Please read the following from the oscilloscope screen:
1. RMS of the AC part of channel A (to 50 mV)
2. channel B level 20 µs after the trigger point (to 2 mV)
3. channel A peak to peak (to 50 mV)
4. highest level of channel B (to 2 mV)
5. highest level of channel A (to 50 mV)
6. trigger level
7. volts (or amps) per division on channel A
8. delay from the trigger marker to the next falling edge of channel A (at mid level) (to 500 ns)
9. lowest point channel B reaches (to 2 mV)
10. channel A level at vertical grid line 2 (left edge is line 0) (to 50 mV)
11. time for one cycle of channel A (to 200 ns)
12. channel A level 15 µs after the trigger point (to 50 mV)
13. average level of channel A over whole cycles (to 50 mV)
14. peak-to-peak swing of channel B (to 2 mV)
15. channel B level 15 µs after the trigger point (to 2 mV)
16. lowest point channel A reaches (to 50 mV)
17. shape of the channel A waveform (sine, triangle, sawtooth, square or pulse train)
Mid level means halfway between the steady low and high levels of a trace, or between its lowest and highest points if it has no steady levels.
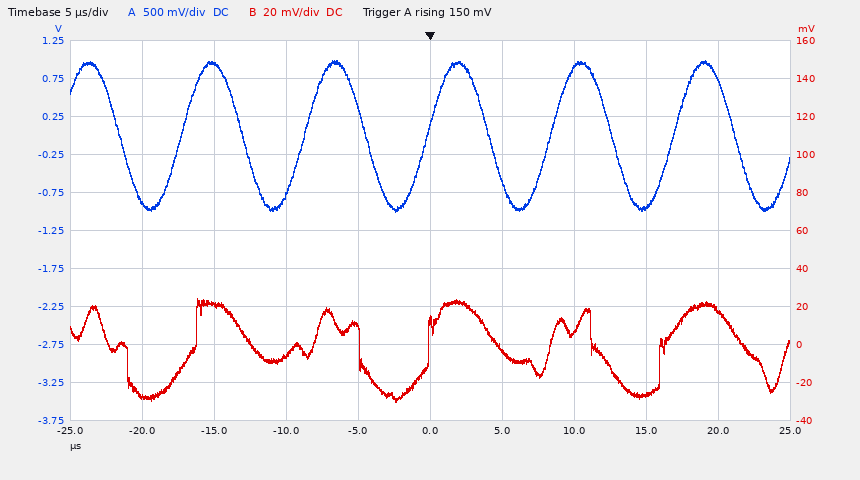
700 mV
18 mV
2.00 V
24 mV
1.00 V
150 mV
500 mV
4.0 µs
-30 mV
950 mV
8.6 µs
-950 mV
0 mV
54 mV
-26 mV
-1.00 V
sine
